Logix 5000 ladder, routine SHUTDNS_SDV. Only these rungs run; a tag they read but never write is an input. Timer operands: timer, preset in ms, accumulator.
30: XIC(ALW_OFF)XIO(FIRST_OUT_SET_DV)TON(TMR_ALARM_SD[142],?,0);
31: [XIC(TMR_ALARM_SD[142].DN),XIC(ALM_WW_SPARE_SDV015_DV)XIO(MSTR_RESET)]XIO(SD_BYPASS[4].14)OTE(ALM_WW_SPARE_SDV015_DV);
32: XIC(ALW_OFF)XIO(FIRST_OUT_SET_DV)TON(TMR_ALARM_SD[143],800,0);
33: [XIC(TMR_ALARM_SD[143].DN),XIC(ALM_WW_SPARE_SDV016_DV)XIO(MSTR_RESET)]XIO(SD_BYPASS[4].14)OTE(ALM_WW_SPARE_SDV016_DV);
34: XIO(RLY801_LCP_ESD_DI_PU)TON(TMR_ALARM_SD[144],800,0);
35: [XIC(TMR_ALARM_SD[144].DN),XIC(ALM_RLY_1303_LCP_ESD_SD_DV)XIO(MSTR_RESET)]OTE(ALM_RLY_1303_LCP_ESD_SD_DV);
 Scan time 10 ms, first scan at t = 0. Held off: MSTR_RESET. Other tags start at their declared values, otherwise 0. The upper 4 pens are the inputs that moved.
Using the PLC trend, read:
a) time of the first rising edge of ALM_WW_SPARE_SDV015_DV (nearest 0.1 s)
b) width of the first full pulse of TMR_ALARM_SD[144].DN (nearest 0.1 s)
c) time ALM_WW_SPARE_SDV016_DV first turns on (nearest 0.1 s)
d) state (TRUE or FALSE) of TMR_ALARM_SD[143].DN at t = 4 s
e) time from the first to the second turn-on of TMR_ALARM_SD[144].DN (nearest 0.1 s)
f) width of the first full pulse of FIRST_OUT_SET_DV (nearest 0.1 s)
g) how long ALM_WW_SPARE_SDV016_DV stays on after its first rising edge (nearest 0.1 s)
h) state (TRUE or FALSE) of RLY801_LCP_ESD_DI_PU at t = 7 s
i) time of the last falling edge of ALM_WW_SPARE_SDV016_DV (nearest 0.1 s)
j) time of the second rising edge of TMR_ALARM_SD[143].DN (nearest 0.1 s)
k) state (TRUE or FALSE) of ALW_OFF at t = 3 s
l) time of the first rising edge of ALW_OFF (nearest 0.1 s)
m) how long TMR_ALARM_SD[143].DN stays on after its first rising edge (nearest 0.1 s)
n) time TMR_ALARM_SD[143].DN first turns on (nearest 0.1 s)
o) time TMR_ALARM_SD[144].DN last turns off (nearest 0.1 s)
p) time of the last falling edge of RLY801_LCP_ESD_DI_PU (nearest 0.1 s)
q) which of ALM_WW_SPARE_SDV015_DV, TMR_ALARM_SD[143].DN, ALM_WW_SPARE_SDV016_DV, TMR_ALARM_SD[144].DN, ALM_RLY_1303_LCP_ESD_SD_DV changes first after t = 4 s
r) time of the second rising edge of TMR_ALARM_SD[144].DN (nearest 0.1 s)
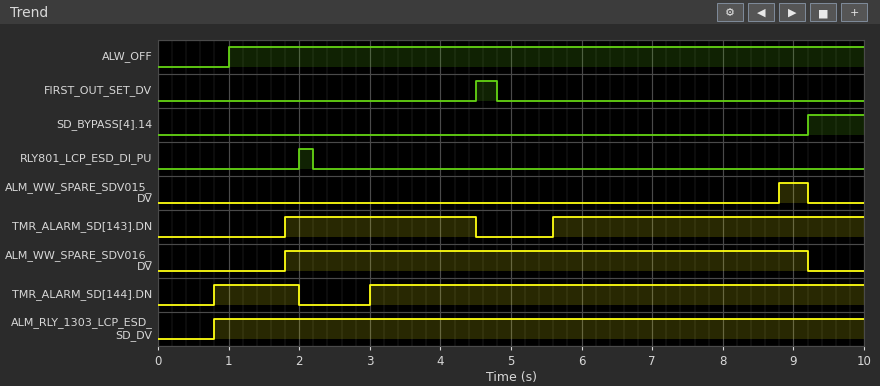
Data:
8.8 s
1.2 s
1.8 s
TRUE
2.2 s
0.3 s
7.4 s
FALSE
9.2 s
5.6 s
TRUE
1.0 s
2.7 s
1.8 s
2.0 s
2.2 s
TMR_ALARM_SD[143].DN
3.0 s
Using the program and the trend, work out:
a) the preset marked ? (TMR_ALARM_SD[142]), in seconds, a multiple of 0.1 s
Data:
4.0 s
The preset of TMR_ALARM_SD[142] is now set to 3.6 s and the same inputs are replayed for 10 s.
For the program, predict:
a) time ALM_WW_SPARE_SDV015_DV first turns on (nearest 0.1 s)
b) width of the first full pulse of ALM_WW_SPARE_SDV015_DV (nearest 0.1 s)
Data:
8.4 s
0.8 s
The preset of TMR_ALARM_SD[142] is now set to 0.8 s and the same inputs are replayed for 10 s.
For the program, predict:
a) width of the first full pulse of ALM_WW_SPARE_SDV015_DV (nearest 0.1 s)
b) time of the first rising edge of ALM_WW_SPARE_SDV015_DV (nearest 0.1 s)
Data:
7.4 s
1.8 s
